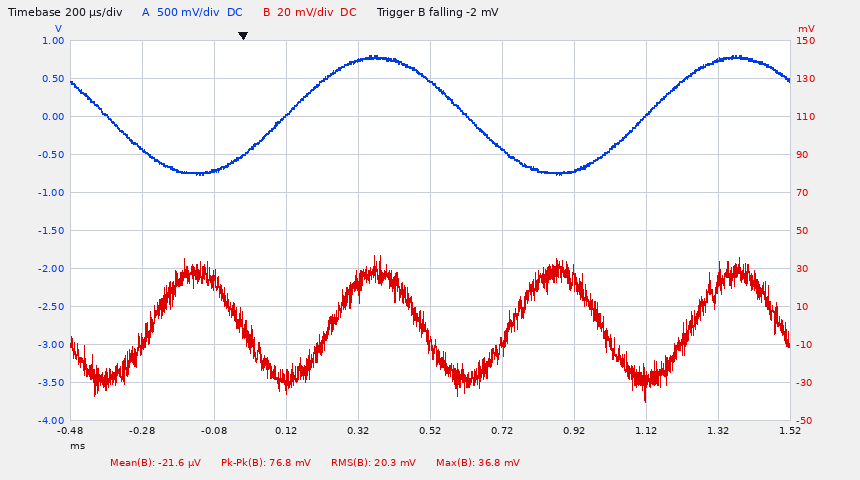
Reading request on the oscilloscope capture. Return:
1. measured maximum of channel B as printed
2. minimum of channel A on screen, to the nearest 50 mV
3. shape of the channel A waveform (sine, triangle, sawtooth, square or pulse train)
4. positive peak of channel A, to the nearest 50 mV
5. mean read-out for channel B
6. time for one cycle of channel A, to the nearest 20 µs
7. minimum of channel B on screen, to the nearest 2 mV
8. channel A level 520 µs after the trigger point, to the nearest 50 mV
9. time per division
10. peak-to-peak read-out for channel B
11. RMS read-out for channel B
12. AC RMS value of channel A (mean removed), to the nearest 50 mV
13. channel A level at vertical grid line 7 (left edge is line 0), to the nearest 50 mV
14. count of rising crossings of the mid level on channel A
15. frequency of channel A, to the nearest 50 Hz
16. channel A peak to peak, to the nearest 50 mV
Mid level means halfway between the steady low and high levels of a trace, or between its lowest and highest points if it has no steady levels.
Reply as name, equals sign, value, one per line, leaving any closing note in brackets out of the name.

measured maximum of channel B as printed = 36.8 mV
minimum of channel A on screen, to the nearest 50 mV = -750 mV
shape of the channel A waveform = sine
positive peak of channel A, to the nearest 50 mV = 800 mV
mean read-out for channel B = -21.6 µV
time for one cycle of channel A, to the nearest 20 µs = 1.00 ms
minimum of channel B on screen, to the nearest 2 mV = -40 mV
channel A level 520 µs after the trigger point, to the nearest 50 mV = 450 mV
time per division = 200 µs
peak-to-peak read-out for channel B = 76.8 mV
RMS read-out for channel B = 20.3 mV
AC RMS value of channel A (mean removed), to the nearest 50 mV = 550 mV
channel A level at vertical grid line 7 (left edge is line 0), to the nearest 50 mV = -700 mV
count of rising crossings of the mid level on channel A = 2
frequency of channel A, to the nearest 50 Hz = 1.00 kHz
channel A peak to peak, to the nearest 50 mV = 1.55 V
